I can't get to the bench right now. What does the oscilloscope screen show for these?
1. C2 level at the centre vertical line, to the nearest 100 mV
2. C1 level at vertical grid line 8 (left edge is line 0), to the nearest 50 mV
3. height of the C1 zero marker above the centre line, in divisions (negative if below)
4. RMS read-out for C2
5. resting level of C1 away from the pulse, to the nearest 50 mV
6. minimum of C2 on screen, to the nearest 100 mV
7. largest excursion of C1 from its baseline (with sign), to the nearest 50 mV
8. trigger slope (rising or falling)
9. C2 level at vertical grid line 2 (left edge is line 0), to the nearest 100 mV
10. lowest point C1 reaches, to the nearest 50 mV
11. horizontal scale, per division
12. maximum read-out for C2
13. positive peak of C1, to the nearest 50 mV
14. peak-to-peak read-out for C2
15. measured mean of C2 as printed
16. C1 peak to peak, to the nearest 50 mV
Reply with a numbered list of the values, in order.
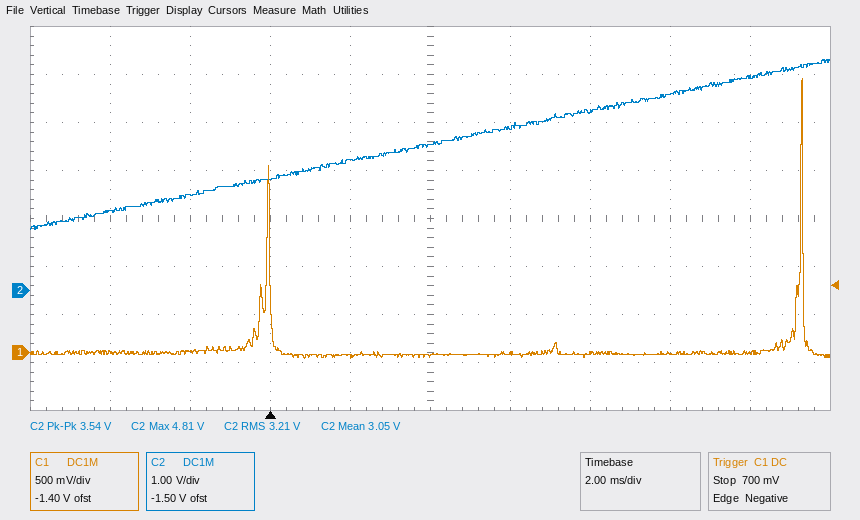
1. 3.0 V
2. 0 mV
3. -2.8 div
4. 3.21 V
5. 0 mV
6. 1.3 V
7. +2.85 V
8. falling
9. 2.0 V
10. -50 mV
11. 2 ms
12. 4.81 V
13. 2.85 V
14. 3.54 V
15. 3.05 V
16. 2.90 V
